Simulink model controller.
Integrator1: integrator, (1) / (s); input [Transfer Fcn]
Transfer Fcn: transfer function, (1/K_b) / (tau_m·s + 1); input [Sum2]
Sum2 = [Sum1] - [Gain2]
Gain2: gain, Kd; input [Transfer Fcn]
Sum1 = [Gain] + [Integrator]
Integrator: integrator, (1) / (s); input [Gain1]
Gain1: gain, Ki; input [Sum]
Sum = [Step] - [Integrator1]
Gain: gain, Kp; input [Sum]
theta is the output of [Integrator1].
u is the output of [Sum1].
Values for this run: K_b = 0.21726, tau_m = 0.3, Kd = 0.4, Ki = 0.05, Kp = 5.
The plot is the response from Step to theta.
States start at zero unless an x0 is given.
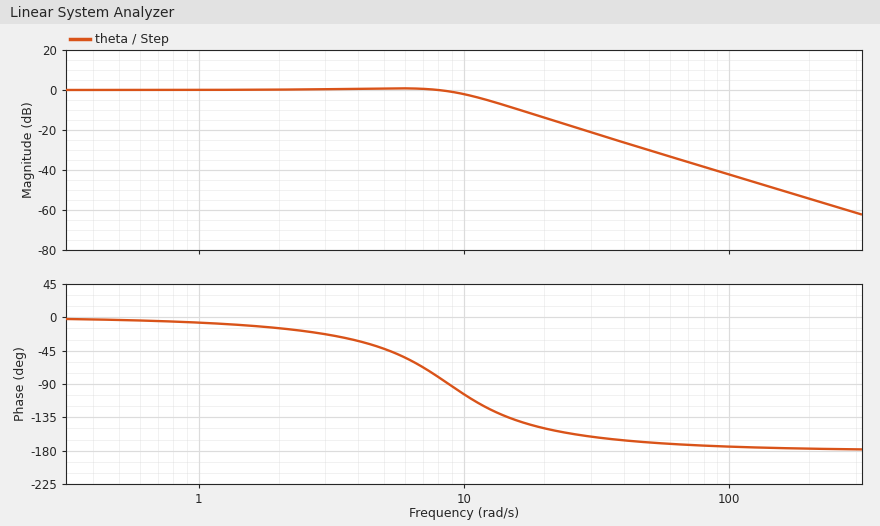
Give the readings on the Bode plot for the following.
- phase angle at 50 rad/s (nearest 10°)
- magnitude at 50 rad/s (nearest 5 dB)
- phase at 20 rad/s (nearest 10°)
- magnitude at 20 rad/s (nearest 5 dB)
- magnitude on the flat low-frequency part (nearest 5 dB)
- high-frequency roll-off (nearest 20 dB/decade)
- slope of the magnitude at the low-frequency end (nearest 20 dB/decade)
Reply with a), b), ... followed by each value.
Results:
a) -170°
b) -30 dB
c) -150°
d) -15 dB
e) 0 dB
f) -40 dB/decade
g) 0 dB/decade
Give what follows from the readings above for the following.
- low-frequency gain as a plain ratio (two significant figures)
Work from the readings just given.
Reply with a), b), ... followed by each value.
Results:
a) 1.0
